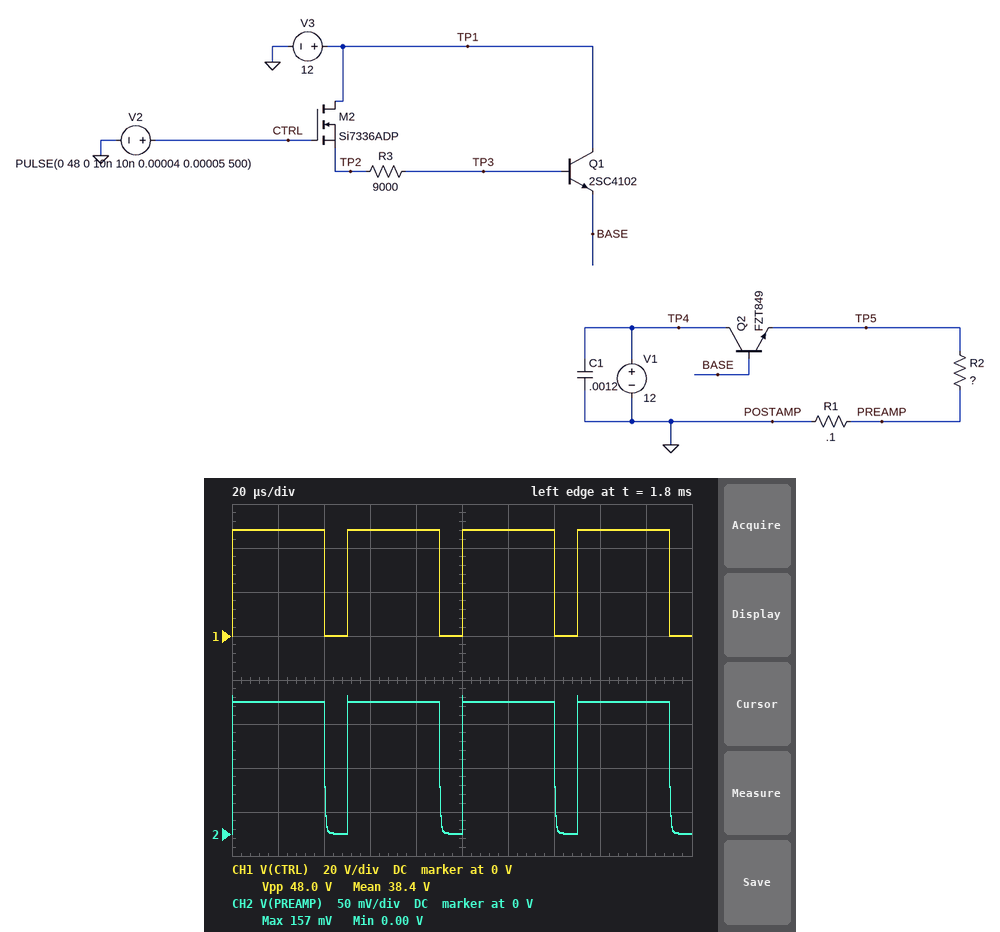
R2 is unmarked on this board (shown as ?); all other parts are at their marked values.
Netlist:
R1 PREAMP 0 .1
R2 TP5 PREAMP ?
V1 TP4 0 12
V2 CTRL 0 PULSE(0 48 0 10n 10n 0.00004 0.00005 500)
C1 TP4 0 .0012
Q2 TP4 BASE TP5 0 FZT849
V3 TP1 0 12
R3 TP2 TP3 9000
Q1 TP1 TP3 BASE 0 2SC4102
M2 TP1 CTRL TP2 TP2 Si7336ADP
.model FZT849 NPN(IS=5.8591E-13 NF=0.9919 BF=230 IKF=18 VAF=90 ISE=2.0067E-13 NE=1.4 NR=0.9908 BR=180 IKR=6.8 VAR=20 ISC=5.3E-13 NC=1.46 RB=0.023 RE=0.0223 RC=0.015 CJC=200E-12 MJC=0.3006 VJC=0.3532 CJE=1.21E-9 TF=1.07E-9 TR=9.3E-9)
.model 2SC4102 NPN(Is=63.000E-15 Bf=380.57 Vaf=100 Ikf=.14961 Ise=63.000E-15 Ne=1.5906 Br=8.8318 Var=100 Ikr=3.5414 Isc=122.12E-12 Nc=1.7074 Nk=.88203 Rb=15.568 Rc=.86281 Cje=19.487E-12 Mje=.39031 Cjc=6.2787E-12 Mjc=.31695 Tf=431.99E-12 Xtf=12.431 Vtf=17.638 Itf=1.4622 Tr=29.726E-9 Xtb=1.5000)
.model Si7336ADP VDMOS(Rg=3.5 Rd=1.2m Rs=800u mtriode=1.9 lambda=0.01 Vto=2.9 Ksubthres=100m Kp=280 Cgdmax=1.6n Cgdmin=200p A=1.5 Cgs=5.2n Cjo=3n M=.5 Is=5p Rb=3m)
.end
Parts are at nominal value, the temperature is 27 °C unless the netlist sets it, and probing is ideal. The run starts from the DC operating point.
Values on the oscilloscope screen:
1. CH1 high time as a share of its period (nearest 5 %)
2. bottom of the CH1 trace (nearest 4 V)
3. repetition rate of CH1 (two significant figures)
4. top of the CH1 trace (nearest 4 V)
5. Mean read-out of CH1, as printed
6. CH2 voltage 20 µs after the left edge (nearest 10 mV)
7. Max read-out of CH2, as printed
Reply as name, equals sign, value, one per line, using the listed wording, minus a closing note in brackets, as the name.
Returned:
CH1 high time as a share of its period = 80 %
bottom of the CH1 trace = 0 V
repetition rate of CH1 = 20 kHz
top of the CH1 trace = 48 V
Mean read-out of CH1, as printed = 38.4 V
CH2 voltage 20 µs after the left edge = 150 mV
Max read-out of CH2, as printed = 157 mV
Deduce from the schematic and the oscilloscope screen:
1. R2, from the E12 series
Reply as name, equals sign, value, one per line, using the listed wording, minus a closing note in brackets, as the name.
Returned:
R2, from the E12 series = 6.8 Ω
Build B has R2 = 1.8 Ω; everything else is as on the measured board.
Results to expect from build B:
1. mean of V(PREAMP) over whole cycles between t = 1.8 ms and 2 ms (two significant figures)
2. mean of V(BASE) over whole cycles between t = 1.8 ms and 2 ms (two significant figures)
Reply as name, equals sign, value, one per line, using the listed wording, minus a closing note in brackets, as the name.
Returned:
mean of V(PREAMP) over whole cycles between t = 1.8 ms and 2 ms = 400 mV
mean of V(BASE) over whole cycles between t = 1.8 ms and 2 ms = 8.4 V
